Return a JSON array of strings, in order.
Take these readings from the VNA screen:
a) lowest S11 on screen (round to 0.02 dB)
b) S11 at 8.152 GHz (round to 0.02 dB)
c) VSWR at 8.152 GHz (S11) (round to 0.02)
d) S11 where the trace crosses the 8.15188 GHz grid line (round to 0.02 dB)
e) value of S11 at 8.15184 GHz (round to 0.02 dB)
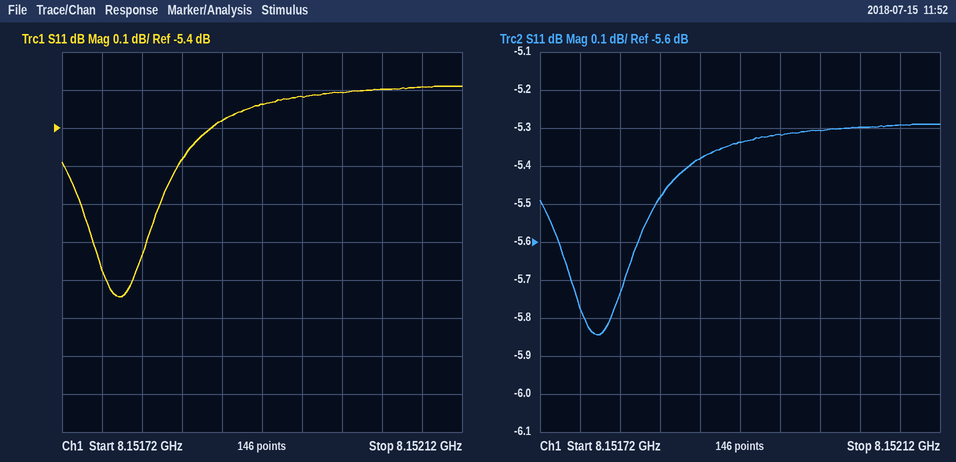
["-5.84 dB", "-5.30 dB", "3.38", "-5.38 dB", "-5.48 dB"]
